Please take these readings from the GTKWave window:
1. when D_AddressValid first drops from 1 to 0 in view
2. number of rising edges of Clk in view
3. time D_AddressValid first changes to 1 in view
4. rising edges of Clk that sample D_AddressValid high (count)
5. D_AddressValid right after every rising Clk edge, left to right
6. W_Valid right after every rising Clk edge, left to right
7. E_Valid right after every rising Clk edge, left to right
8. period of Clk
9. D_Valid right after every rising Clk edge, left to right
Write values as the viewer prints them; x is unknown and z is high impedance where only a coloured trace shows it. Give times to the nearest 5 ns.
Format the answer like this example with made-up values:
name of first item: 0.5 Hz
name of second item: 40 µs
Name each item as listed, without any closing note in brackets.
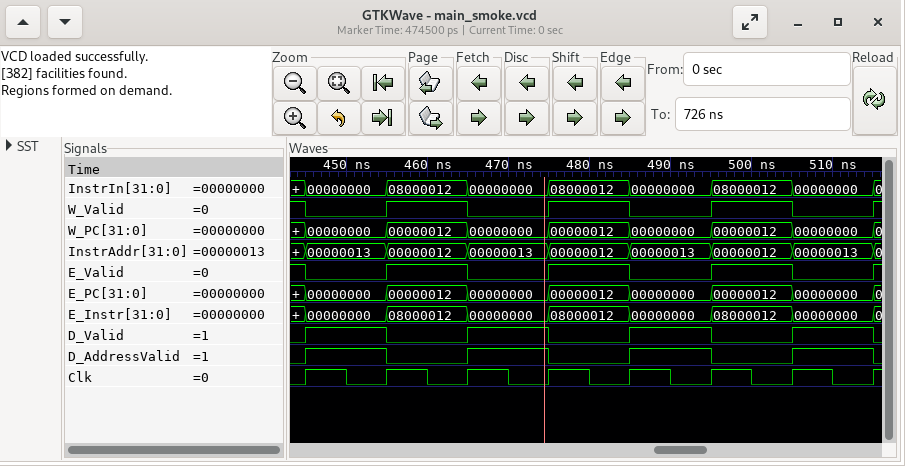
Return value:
when D_AddressValid first drops from 1 to 0 in view: 455 ns
number of rising edges of Clk in view: 8
time D_AddressValid first changes to 1 in view: 445 ns
rising edges of Clk that sample D_AddressValid high: 4
D_AddressValid right after every rising Clk edge, left to right: 1 0 1 0 1 0 1 0
W_Valid right after every rising Clk edge, left to right: 0 1 0 1 0 1 0 1
E_Valid right after every rising Clk edge, left to right: 0 1 0 1 0 1 0 1
period of Clk: 10 ns
D_Valid right after every rising Clk edge, left to right: 1 0 1 0 1 0 1 0
